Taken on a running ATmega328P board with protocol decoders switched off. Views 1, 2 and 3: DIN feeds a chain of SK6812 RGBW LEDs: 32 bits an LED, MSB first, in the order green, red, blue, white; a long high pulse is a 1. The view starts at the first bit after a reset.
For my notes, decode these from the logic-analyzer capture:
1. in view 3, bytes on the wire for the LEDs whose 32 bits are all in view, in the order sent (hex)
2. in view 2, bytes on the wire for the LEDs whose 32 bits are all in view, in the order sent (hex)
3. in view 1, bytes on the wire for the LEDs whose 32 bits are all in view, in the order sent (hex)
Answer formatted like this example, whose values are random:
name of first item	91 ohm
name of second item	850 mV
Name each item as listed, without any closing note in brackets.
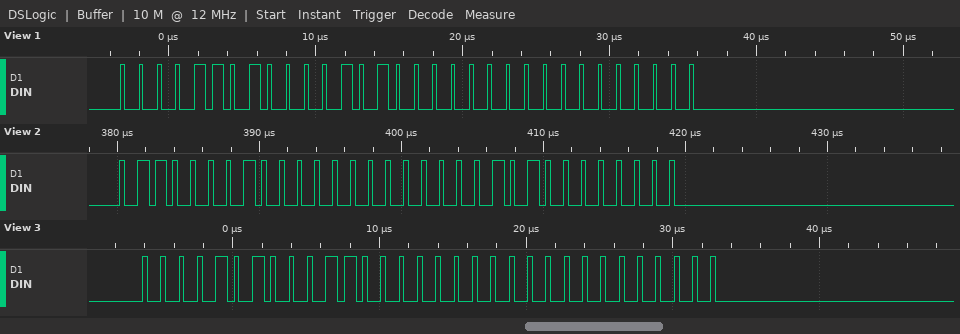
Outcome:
in view 3, bytes on the wire for the LEDs whose 32 bits are all in view, in the order sent	0A 30 00 00
in view 2, bytes on the wire for the LEDs whose 32 bits are all in view, in the order sent	61 00 05 00
in view 1, bytes on the wire for the LEDs whose 32 bits are all in view, in the order sent	0D 0A 00 00
